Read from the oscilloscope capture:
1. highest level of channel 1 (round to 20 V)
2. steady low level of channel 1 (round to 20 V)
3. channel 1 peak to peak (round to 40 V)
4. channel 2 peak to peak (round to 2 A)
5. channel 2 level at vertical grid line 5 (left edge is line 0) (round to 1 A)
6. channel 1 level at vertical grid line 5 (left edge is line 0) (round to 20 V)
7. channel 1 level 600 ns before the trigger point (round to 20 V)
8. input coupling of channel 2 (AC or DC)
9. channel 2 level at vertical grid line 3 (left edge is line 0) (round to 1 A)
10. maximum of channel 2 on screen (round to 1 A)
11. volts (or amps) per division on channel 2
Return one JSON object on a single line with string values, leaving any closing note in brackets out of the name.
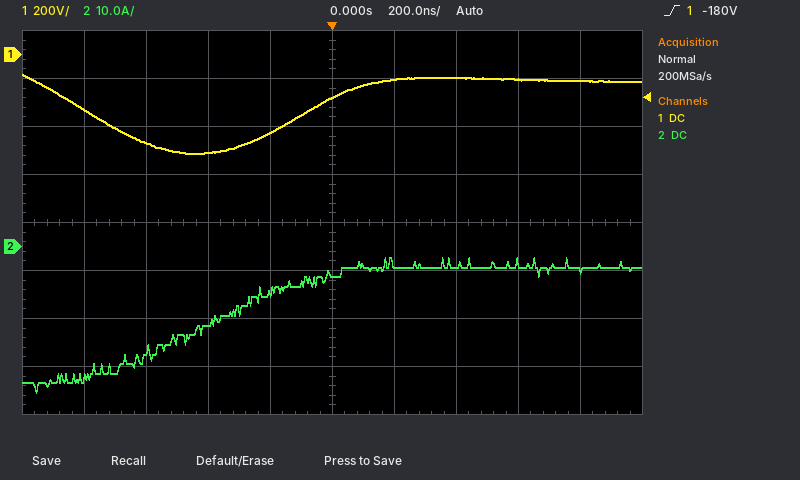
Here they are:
{"highest level of channel 1": "-80 V", "steady low level of channel 1": "-400 V", "channel 1 peak to peak": "320 V", "channel 2 peak to peak": "28 A", "channel 2 level at vertical grid line 5 (left edge is line 0)": "-6 A", "channel 1 level at vertical grid line 5 (left edge is line 0)": "-180 V", "channel 1 level 600 ns before the trigger point": "-360 V", "input coupling of channel 2": "DC", "channel 2 level at vertical grid line 3 (left edge is line 0)": "-16 A", "maximum of channel 2 on screen": "-2 A", "volts (or amps) per division on channel 2": "10 A"}
